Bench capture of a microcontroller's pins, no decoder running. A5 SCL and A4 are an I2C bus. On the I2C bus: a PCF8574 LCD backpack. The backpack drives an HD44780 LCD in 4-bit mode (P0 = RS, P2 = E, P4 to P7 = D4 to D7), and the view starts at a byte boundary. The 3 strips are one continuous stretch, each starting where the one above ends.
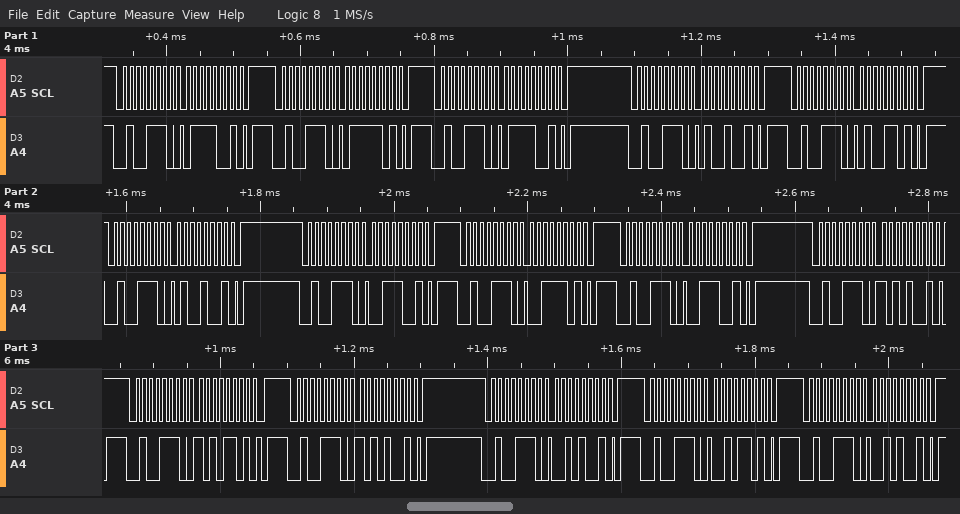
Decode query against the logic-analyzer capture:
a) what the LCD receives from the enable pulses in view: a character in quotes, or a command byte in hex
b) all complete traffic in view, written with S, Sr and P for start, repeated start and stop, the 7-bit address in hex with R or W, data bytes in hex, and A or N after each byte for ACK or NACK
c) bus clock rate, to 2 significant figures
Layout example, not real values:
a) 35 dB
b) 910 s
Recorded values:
a) 't' ':'
b) S 27W A 79 A P S 27W A 7D A P S 27W A 79 A P S 27W A 49 A P S 27W A 4D A P S 27W A 49 A P S 27W A 39 A P S 27W A 3D A P S 27W A 39 A P S 27W A A9 A P S 27W A AD A P S 27W A A9 A P S 27W A 29 A P S 27W A 2D A P S 27W A 29 A P
c) 100 kHz
